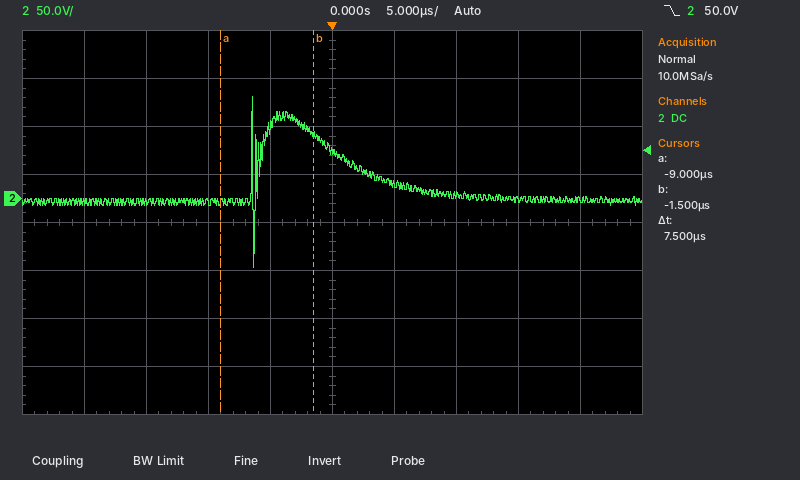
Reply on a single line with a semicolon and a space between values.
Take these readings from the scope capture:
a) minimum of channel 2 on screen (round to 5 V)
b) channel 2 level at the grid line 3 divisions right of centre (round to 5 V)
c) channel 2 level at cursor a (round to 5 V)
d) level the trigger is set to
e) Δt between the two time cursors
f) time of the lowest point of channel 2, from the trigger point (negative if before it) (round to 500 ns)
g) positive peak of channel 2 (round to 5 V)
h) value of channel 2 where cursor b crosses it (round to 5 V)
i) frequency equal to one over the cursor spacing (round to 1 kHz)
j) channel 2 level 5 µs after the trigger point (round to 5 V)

-70 V; 0 V; -5 V; 50.0 V; 7.5 µs; -6.5 µs; 105 V; 65 V; 133 kHz; 15 V
